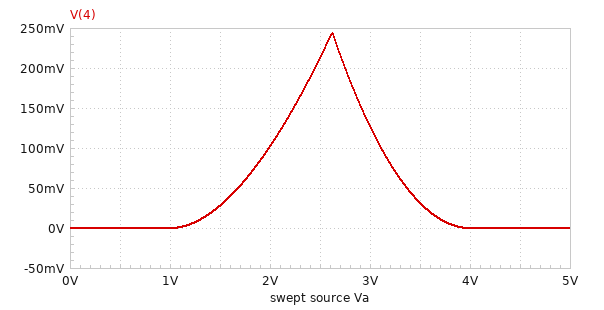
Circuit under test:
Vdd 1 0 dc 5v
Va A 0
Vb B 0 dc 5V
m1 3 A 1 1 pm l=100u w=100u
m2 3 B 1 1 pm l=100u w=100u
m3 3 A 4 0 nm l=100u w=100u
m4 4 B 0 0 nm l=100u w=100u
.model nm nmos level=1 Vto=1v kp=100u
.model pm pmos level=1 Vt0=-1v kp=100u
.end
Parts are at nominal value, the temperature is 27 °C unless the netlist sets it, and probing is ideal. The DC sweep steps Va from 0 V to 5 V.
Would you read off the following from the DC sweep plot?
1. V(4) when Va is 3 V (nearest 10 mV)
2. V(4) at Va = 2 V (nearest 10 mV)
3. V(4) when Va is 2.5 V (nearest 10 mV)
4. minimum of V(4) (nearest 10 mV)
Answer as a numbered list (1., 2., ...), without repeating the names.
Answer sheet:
1. 130 mV
2. 100 mV
3. 210 mV
4. 0 V
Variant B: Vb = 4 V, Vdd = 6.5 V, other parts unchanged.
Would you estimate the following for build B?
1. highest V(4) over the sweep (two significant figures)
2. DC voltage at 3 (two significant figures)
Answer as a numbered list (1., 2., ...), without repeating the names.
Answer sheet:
1. 880 mV
2. 6.5 V
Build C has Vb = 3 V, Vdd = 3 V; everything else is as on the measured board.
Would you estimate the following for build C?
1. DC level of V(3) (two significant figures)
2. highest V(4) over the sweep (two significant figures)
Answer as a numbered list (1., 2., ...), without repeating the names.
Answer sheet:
1. 3.0 V
2. 56 mV
